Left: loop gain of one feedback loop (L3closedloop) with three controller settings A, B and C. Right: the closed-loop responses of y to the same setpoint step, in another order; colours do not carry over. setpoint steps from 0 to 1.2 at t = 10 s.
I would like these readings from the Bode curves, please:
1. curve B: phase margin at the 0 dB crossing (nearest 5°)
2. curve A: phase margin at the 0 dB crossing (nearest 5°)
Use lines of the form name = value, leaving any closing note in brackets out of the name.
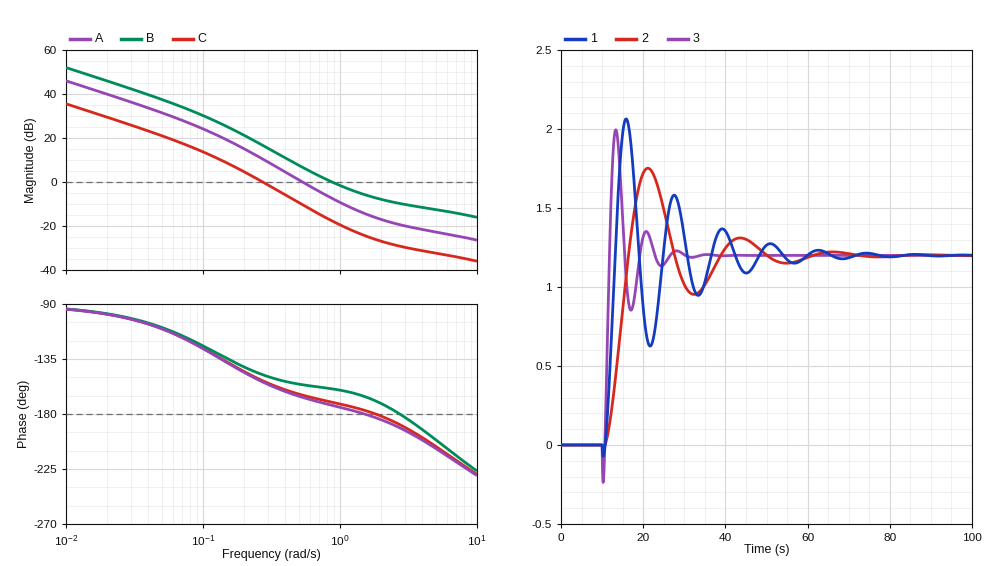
curve B: phase margin at the 0 dB crossing = 20°
curve A: phase margin at the 0 dB crossing = 15°
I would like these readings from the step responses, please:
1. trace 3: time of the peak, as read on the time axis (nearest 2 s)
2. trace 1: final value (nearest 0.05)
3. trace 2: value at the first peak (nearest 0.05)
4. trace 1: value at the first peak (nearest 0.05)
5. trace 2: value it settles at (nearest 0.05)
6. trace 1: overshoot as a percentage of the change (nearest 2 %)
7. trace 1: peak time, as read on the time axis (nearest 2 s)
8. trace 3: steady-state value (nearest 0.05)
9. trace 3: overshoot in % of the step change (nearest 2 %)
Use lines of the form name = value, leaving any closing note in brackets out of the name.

trace 3: time of the peak, as read on the time axis = 14 s
trace 1: final value = 1.20
trace 2: value at the first peak = 1.75
trace 1: value at the first peak = 2.05
trace 2: value it settles at = 1.20
trace 1: overshoot as a percentage of the change = 72 %
trace 1: peak time, as read on the time axis = 16 s
trace 3: steady-state value = 1.20
trace 3: overshoot in % of the step change = 66 %
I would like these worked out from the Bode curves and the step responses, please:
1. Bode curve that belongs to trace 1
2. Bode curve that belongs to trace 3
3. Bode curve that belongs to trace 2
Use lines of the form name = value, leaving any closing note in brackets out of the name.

Bode curve that belongs to trace 1 = A
Bode curve that belongs to trace 3 = B
Bode curve that belongs to trace 2 = C
